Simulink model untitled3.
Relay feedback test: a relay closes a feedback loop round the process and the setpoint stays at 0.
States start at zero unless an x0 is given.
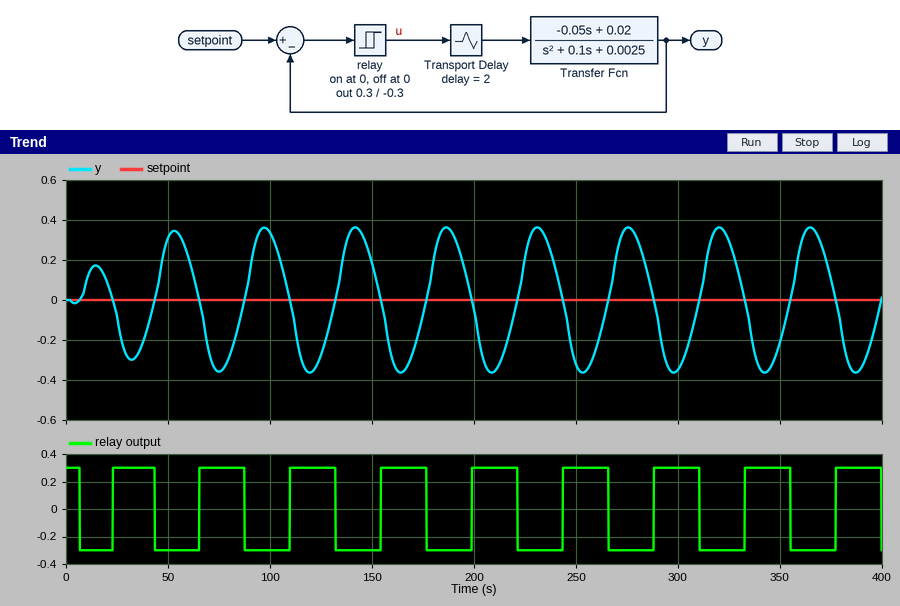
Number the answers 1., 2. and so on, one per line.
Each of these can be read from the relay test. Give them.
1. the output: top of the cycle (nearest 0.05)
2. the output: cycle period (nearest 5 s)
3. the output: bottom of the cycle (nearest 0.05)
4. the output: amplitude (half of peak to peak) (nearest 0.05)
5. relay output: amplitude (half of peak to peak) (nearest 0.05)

1. 0.35
2. 45 s
3. -0.35
4. 0.35
5. 0.30
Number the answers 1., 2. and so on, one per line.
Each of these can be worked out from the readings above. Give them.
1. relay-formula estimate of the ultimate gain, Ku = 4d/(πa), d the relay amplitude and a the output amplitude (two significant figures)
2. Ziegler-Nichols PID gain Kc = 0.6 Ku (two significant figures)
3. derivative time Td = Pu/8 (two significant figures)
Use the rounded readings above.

1. 1.1
2. 0.66
3. 5.6 s
